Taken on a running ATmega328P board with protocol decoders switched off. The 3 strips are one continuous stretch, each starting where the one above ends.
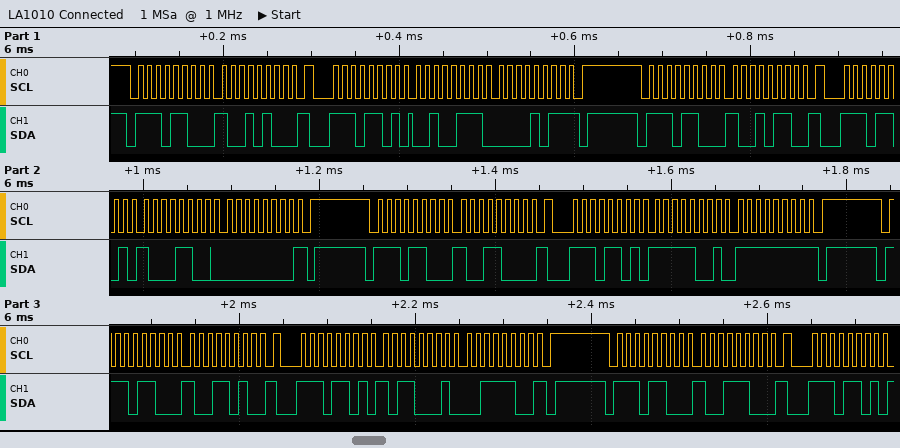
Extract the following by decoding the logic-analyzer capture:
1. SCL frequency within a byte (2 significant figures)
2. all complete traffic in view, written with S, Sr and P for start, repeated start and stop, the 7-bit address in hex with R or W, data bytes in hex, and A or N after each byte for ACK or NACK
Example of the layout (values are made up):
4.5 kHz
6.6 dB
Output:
100 kHz
S 76W A 94 A Sr 76R A 27 A 0B N P S 76W A 96 A Sr 76R A 8C A 00 N P S 76W A 98 A Sr 76R A F9 A FF N P S 76W A 9A A Sr 76R A B1 A 3C N P S 76W A 9C A Sr 76R A
